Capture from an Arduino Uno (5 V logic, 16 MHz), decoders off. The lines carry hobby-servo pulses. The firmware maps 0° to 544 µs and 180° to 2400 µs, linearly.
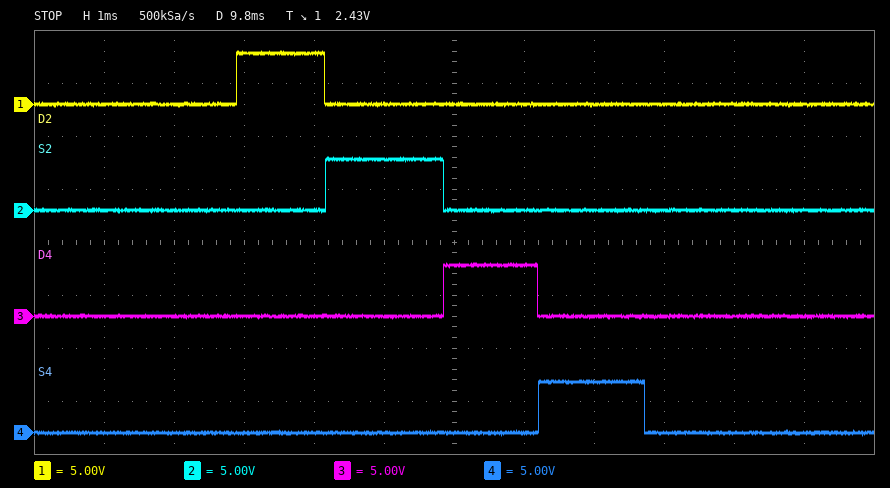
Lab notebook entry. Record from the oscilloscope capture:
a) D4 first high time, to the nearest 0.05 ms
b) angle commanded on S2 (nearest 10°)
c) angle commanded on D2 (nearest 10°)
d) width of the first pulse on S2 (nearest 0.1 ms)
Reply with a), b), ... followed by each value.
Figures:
a) 1.35 ms
b) 110°
c) 70°
d) 1.7 ms
